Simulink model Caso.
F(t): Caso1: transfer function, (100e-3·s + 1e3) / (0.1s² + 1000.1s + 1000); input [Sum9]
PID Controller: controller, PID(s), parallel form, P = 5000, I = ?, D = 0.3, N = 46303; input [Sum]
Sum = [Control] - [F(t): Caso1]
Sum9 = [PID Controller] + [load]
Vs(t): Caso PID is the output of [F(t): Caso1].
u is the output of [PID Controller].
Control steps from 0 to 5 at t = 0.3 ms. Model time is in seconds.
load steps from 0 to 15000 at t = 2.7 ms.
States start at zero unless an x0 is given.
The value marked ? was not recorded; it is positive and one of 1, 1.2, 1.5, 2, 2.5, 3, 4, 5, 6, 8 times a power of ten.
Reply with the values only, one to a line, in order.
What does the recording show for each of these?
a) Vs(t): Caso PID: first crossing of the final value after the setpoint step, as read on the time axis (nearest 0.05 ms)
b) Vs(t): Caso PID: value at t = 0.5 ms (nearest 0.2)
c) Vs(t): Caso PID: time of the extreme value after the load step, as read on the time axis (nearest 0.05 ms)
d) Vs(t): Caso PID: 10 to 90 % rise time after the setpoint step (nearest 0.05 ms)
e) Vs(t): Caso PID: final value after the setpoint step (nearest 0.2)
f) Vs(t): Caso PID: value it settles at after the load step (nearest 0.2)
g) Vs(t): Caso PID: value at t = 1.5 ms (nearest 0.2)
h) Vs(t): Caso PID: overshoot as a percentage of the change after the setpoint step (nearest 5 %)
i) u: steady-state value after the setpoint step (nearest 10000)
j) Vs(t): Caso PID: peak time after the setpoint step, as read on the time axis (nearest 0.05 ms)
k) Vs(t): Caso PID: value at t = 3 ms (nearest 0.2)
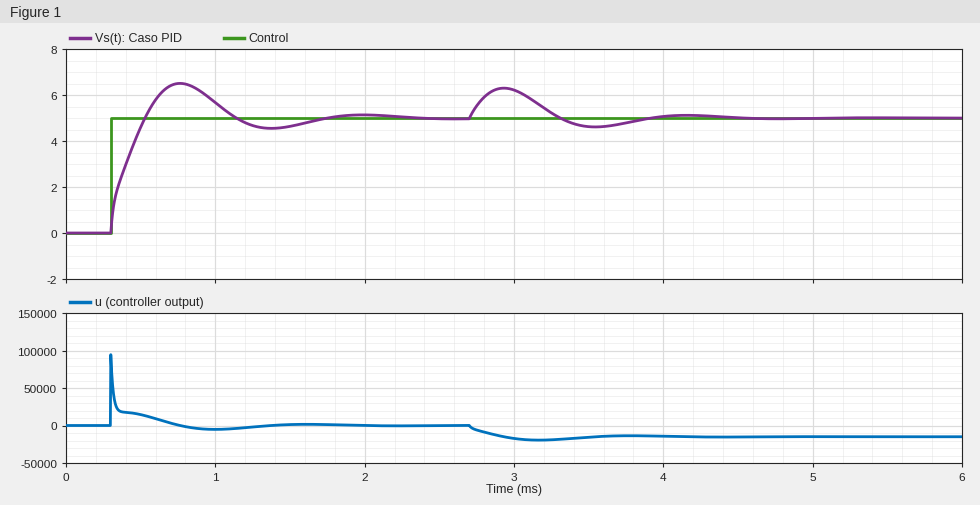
0.55 ms
4.6
2.95 ms
0.20 ms
5.0
5.0
4.6
30 %
0
0.75 ms
6.2
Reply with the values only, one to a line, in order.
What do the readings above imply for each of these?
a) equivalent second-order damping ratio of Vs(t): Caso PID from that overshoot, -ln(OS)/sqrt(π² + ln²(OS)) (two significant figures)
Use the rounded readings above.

0.36
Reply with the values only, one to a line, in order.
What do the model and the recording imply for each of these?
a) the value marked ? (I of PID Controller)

4e+07
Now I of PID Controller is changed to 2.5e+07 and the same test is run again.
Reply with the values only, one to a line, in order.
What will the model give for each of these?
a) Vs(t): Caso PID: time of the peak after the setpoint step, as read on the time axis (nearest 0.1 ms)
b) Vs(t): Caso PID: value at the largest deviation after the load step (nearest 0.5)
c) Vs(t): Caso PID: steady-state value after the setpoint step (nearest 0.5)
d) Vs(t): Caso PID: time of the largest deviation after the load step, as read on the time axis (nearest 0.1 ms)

0.9 ms
6.5
5.0
3.0 ms
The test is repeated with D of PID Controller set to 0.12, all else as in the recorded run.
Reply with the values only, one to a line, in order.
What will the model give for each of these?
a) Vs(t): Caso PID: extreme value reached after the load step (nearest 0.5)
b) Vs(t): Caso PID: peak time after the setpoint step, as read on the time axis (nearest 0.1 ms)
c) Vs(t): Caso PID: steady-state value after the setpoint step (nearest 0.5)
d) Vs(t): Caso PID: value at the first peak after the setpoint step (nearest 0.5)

6.5
0.7 ms
5.0
6.5
